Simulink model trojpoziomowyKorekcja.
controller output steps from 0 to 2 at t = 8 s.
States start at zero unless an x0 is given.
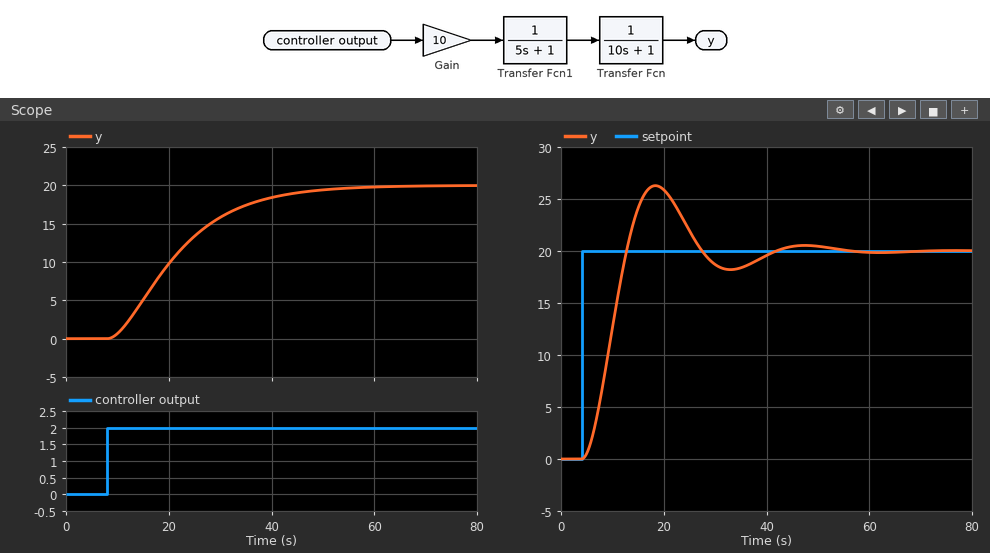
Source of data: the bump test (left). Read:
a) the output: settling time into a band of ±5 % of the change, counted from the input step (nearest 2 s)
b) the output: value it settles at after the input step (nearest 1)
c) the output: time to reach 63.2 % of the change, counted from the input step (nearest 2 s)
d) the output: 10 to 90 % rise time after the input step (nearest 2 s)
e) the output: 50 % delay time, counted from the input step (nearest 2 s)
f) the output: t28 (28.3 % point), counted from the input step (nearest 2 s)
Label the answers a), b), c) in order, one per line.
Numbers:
a) 36 s
b) 20
c) 16 s
d) 26 s
e) 12 s
f) 8 s
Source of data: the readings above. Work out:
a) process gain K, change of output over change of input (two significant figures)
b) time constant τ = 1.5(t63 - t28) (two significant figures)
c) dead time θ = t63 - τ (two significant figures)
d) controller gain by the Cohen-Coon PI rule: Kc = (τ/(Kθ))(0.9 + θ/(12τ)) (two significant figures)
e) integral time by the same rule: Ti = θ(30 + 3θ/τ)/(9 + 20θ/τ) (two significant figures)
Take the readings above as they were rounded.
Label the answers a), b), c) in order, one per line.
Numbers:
a) 10
b) 12 s
c) 4.0 s
d) 0.28
e) 7.9 s
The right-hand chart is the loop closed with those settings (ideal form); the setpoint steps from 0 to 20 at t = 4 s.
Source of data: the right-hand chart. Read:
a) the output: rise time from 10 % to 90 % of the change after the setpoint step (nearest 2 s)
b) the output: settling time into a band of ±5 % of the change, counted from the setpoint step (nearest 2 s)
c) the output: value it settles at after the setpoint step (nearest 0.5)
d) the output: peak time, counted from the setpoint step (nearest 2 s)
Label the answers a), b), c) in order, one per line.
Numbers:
a) 6 s
b) 34 s
c) 20.0
d) 14 s
